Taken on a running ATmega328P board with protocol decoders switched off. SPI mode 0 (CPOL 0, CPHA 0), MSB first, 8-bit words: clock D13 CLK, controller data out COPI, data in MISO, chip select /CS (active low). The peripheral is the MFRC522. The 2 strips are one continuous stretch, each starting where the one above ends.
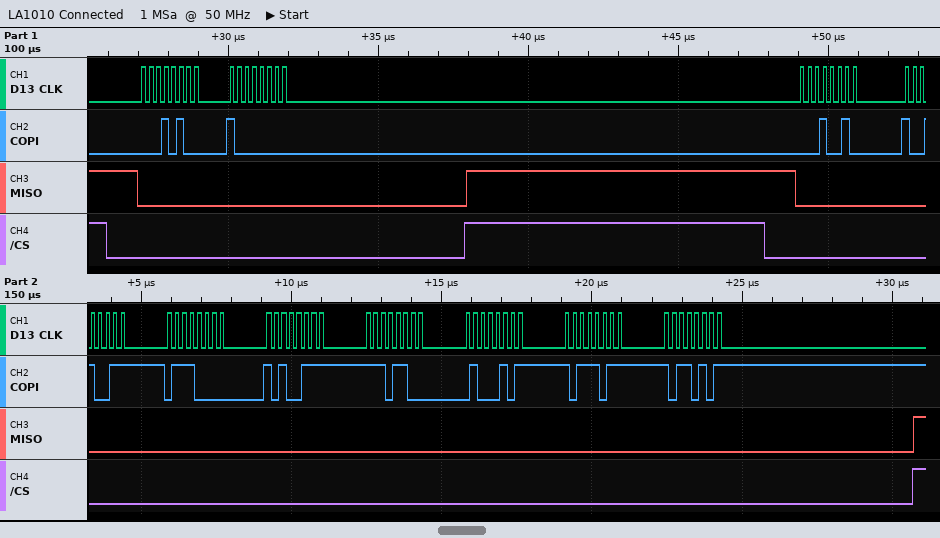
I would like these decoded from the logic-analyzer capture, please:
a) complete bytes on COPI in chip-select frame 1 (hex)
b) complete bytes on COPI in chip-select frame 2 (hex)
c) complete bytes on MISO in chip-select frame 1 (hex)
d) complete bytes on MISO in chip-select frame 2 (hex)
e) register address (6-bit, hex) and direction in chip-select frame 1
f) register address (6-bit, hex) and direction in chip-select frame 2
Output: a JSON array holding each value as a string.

["0x14 0x80", "0x12 0x93 0x70 0xA7 0xEC 0x45 0xBB 0xB5", "0x00 0x00", "0x00 0x00 0x00 0x00 0x00 0x00 0x00 0x00", "0x0A write", "0x09 write"]
